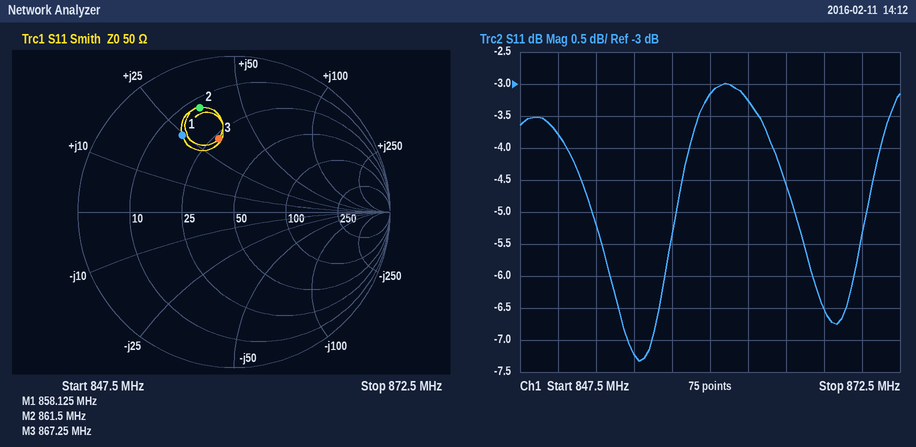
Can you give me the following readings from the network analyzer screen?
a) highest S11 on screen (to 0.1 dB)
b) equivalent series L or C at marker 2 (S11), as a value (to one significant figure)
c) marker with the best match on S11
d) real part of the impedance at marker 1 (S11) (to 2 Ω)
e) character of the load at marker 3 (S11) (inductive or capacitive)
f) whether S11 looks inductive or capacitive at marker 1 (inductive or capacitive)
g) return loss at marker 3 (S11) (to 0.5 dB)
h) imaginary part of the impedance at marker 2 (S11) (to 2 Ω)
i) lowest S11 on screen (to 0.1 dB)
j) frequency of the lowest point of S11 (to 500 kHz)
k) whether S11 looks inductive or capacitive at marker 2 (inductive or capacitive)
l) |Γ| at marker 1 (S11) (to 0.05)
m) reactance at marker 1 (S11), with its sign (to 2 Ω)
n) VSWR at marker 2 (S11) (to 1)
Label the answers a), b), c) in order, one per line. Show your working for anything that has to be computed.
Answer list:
a) -3.0 dB
b) L = 34 Ω/(2π × 861.5 MHz) ≈ 6 nH
c) marker 3
d) 16 Ω
e) inductive
f) inductive
g) 6.5 dB
h) +34 Ω
i) -7.3 dB
j) 855.5 MHz
k) inductive
l) 0.60
m) +24 Ω
n) 6
